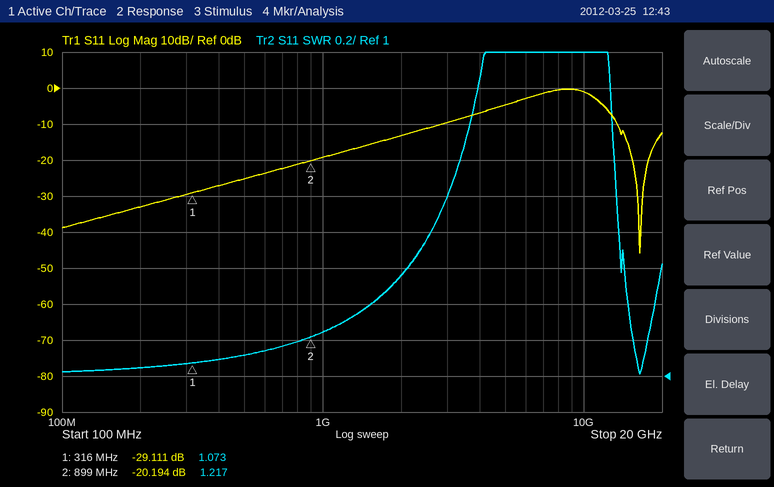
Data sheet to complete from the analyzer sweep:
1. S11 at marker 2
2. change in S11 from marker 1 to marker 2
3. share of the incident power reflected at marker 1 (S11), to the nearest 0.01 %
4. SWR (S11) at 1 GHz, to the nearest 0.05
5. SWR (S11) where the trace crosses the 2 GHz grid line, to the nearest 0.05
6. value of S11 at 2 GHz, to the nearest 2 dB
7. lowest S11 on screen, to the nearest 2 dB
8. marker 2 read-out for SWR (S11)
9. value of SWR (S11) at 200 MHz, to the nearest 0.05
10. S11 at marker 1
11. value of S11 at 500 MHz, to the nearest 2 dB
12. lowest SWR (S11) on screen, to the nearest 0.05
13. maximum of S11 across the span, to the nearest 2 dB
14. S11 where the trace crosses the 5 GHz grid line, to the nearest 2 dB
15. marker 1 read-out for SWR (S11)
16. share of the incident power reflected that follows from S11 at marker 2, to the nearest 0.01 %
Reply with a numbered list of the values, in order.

1. -20.194 dB
2. 8.917 dB
3. 0.12 %
4. 1.25
5. 1.55
6. -14 dB
7. -46 dB
8. 1.217
9. 1.05
10. -29.111 dB
11. -26 dB
12. 1.00
13. 0 dB
14. -4 dB
15. 1.073
16. 0.96 %
